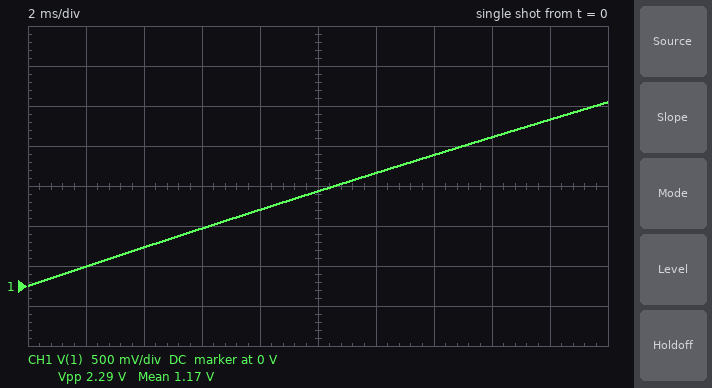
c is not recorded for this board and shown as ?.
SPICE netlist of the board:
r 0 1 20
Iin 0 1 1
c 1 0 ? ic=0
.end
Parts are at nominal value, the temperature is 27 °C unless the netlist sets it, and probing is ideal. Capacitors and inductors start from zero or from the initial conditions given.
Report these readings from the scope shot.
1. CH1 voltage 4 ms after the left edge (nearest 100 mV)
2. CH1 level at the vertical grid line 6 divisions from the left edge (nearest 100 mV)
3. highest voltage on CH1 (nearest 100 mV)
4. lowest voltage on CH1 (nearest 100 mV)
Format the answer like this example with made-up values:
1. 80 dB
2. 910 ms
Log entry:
1. 500 mV
2. 1.4 V
3. 2.3 V
4. 0 V
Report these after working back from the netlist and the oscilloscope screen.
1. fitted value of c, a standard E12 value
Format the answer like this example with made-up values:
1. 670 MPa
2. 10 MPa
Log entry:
1. 8.2 mF
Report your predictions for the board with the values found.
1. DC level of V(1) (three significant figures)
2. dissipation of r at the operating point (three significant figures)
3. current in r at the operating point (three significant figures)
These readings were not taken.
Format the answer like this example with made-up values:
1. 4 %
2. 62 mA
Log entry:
1. 20.0 V
2. 20.0 W
3. 1.00 A
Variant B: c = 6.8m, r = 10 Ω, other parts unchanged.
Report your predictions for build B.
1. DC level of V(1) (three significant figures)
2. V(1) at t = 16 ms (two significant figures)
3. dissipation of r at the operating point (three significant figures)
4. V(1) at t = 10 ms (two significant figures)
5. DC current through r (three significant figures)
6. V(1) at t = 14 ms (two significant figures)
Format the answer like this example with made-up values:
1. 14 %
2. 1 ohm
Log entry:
1. 10.0 V
2. 2.1 V
3. 10.0 W
4. 1.4 V
5. 1.00 A
6. 1.9 V
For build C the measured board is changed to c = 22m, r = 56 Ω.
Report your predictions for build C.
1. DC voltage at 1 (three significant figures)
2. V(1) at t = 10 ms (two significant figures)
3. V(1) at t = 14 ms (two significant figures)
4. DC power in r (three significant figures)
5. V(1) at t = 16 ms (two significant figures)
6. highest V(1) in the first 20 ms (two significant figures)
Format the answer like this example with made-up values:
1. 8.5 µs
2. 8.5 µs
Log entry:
1. 56.0 V
2. 450 mV
3. 630 mV
4. 56.0 W
5. 720 mV
6. 900 mV
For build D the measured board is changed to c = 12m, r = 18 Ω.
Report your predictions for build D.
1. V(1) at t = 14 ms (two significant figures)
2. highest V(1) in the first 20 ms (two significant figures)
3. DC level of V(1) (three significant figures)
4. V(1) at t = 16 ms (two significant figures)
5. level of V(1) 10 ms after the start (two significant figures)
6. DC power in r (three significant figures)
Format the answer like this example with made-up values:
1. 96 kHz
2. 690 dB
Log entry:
1. 1.1 V
2. 1.6 V
3. 18.0 V
4. 1.3 V
5. 810 mV
6. 18.0 W
